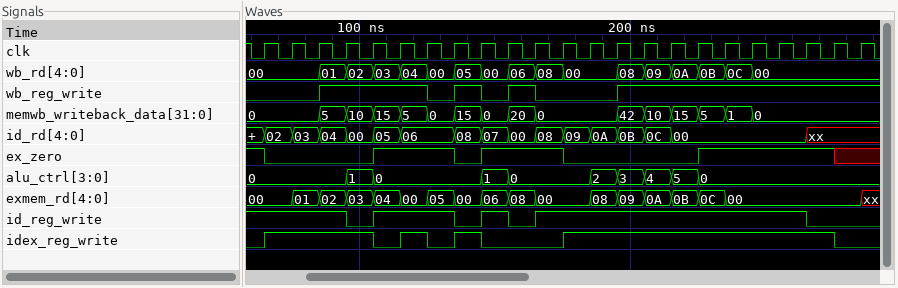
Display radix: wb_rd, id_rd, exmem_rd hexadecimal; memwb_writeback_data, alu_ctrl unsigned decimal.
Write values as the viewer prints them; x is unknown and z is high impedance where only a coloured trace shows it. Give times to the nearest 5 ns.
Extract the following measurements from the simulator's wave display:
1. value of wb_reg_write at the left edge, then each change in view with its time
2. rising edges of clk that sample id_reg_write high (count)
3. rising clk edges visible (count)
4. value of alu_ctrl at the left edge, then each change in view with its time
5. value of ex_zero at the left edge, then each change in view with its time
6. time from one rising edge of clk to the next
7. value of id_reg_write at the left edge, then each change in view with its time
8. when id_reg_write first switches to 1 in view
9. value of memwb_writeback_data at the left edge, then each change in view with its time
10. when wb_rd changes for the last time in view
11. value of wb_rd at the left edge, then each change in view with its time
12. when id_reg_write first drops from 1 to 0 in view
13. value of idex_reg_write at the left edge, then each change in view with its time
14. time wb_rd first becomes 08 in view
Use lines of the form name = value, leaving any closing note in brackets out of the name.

value of wb_reg_write at the left edge, then each change in view with its time = 0, 1 at 85 ns, 0 at 125 ns, 1 at 135 ns, 0 at 145 ns, 1 at 155 ns, 0 at 165 ns, 1 at 195 ns
rising edges of clk that sample id_reg_write high = 18
rising clk edges visible = 23
value of alu_ctrl at the left edge, then each change in view with its time = 0, 1 at 95 ns, 0 at 105 ns, 1 at 145 ns, 0 at 155 ns, 2 at 185 ns, 3 at 195 ns, 4 at 205 ns, 5 at 215 ns, 0 at 225 ns
value of ex_zero at the left edge, then each change in view with its time = 1, 0 at 65 ns, 1 at 105 ns, 0 at 135 ns, 1 at 145 ns, 0 at 175 ns, 1 at 225 ns, x at 275 ns
time from one rising edge of clk to the next = 10 ns
value of id_reg_write at the left edge, then each change in view with its time = 1, 0 at 95 ns, 1 at 105 ns, 0 at 135 ns, 1 at 145 ns, 0 at 155 ns, 1 at 165 ns, 0 at 265 ns
when id_reg_write first switches to 1 in view = 105 ns
value of memwb_writeback_data at the left edge, then each change in view with its time = 0, 5 at 85 ns, 10 at 95 ns, 15 at 105 ns, 5 at 115 ns, 0 at 125 ns, 15 at 135 ns, 0 at 145 ns, 20 at 155 ns, 0 at 165 ns, 42 at 195 ns, 10 at 205 ns, 15 at 215 ns, 5 at 225 ns, 1 at 235 ns, 0 at 245 ns
when wb_rd changes for the last time in view = 245 ns
value of wb_rd at the left edge, then each change in view with its time = 00, 01 at 85 ns, 02 at 95 ns, 03 at 105 ns, 04 at 115 ns, 00 at 125 ns, 05 at 135 ns, 00 at 145 ns, 06 at 155 ns, 08 at 165 ns, 00 at 175 ns, 08 at 195 ns, 09 at 205 ns, 0A at 215 ns, 0B at 225 ns, 0C at 235 ns, 00 at 245 ns
when id_reg_write first drops from 1 to 0 in view = 95 ns
value of idex_reg_write at the left edge, then each change in view with its time = 0, 1 at 65 ns, 0 at 105 ns, 1 at 115 ns, 0 at 125 ns, 1 at 135 ns, 0 at 145 ns, 1 at 175 ns, 0 at 275 ns
time wb_rd first becomes 08 in view = 165 ns
